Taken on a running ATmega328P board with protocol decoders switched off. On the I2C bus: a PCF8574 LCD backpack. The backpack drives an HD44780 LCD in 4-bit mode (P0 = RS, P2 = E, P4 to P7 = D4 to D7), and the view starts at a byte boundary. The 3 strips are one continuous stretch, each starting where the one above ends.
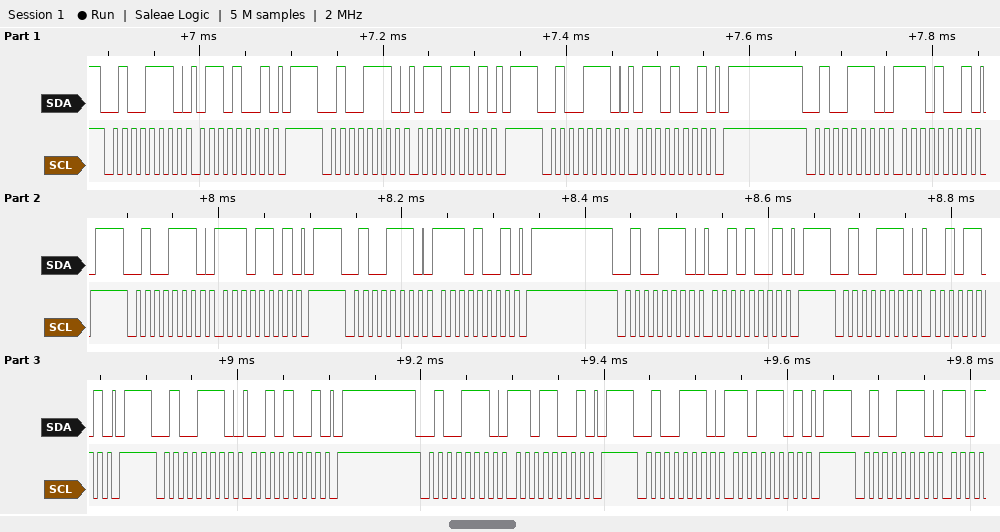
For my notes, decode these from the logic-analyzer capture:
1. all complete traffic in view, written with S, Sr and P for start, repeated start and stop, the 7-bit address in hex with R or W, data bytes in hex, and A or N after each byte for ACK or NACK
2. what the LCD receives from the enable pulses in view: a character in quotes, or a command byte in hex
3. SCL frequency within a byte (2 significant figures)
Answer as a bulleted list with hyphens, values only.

- S 27W A 69 A P S 27W A 6D A P S 27W A 69 A P S 27W A E9 A P S 27W A ED A P S 27W A E9 A P S 27W A 29 A P S 27W A 2D A P S 27W A 29 A P S 27W A D9 A P S 27W A DD A P S 27W A
- 'n'
- 100 kHz
